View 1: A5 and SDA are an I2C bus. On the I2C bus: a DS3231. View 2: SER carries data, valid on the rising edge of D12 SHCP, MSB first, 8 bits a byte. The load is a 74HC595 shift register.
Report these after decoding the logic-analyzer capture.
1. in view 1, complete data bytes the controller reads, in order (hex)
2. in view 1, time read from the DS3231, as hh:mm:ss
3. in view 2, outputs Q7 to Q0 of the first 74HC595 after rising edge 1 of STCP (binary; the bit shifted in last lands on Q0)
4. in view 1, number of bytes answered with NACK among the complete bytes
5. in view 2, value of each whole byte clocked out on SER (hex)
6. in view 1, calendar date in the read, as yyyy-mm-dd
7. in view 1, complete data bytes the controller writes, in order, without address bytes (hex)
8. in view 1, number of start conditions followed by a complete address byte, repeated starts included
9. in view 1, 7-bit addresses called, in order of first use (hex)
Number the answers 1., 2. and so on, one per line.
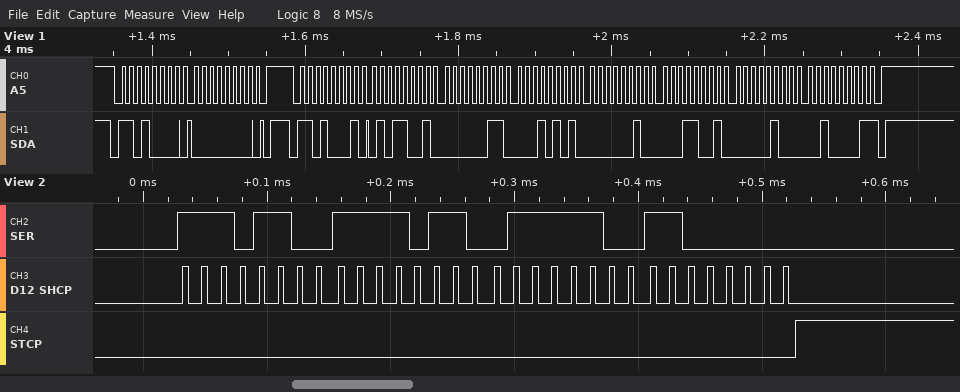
1. 59 03 15 02 19 04 21
2. 15:03:59
3. 11000000
4. 1
5. EC F6 7C C0
6. 2021-04-19
7. 00
8. 2
9. 0x68
